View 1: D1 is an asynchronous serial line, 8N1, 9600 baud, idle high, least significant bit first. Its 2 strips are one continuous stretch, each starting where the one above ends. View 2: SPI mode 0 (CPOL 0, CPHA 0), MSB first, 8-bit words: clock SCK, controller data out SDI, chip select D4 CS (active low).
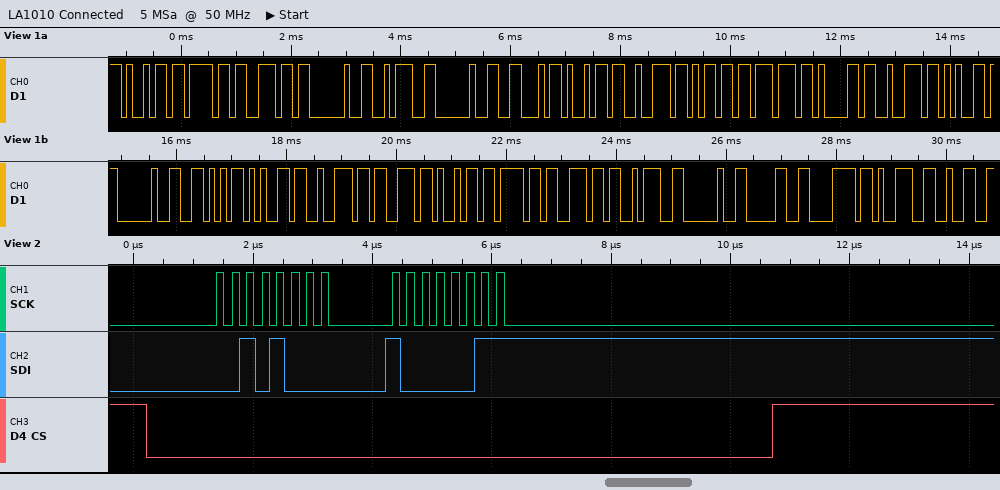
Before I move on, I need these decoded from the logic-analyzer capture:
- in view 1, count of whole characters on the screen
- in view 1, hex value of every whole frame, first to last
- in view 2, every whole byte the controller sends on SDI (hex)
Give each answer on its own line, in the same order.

28
69 6F 6E 20 3A 20 46 69 72 6D 77 61 72 65 20 56 65 72 73 69 6F 6E 3A 20 30 78 39 32
0x28 0x83
